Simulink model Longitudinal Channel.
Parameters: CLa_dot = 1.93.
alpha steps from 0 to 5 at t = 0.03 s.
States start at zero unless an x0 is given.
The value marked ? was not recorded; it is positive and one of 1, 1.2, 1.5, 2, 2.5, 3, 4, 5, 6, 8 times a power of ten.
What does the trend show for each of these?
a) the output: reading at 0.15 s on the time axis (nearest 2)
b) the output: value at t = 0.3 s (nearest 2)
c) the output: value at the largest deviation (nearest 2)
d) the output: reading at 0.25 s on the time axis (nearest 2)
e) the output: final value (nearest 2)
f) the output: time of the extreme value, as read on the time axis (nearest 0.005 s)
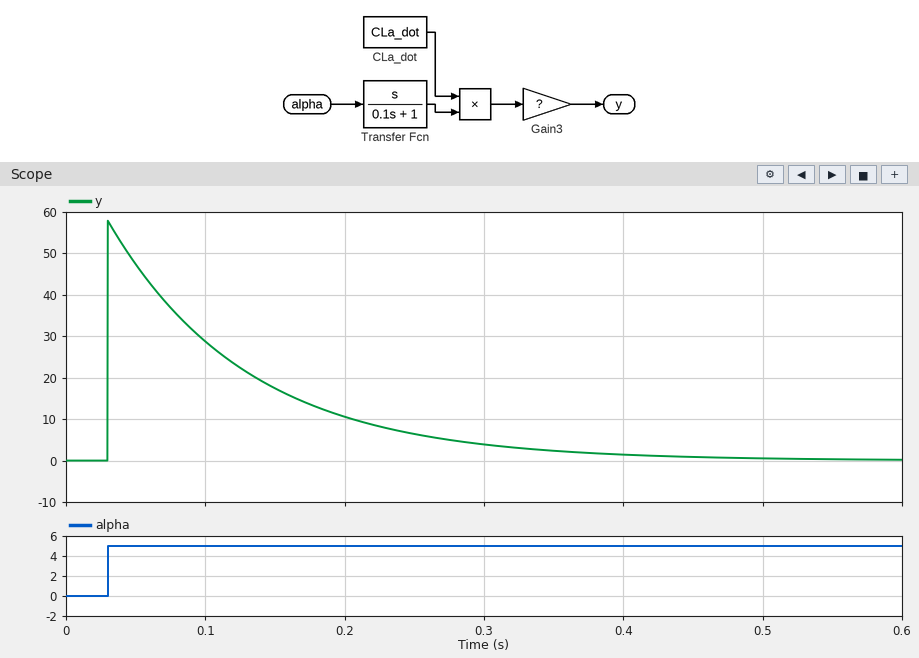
18
4
58
6
0
0.030 s
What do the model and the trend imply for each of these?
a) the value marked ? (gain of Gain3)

0.6
